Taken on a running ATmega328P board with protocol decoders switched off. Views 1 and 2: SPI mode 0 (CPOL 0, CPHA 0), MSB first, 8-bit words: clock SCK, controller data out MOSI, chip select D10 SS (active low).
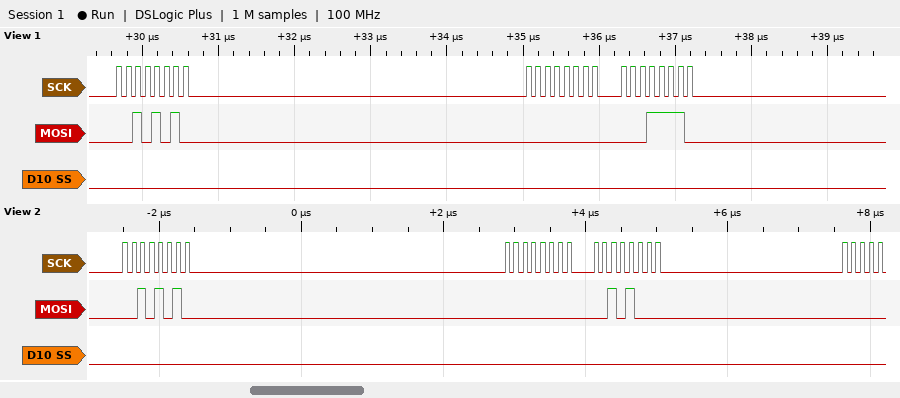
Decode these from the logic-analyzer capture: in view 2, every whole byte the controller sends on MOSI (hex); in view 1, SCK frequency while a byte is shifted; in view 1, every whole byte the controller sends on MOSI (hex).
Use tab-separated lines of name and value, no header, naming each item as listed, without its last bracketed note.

in view 2, every whole byte the controller sends on MOSI	2A 00 28
in view 1, SCK frequency while a byte is shifted	8 MHz
in view 1, every whole byte the controller sends on MOSI	0x2A 0x00 0x1E
